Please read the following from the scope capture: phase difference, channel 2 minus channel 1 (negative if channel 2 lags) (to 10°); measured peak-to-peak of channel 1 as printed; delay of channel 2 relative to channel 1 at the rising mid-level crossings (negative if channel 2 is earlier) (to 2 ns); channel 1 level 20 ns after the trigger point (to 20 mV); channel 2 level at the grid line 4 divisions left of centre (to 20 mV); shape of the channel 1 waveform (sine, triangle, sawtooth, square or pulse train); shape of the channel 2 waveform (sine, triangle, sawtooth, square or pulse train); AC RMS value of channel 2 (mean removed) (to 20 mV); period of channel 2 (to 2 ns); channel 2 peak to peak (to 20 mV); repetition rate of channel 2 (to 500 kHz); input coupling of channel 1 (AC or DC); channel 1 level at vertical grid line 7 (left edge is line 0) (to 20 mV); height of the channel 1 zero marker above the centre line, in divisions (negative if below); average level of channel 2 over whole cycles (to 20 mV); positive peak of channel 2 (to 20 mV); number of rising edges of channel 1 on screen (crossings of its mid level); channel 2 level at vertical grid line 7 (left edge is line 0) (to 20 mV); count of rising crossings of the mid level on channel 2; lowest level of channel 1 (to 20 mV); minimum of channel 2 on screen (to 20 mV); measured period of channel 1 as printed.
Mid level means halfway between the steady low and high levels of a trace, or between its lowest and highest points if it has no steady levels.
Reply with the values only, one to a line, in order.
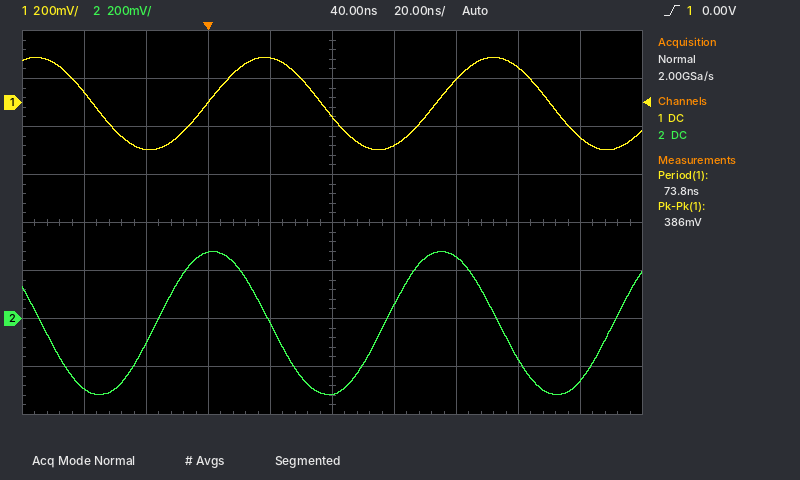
+80°
386 mV
-16 ns
180 mV
-300 mV
sine
sine
220 mV
74 ns
600 mV
13.5 MHz
DC
100 mV
+2.5 div
-20 mV
280 mV
2
260 mV
3
-200 mV
-320 mV
73.8 ns
